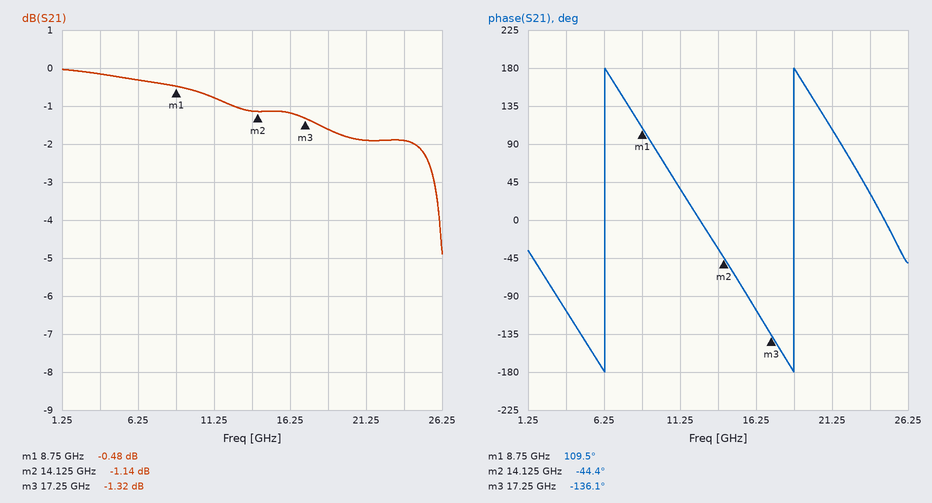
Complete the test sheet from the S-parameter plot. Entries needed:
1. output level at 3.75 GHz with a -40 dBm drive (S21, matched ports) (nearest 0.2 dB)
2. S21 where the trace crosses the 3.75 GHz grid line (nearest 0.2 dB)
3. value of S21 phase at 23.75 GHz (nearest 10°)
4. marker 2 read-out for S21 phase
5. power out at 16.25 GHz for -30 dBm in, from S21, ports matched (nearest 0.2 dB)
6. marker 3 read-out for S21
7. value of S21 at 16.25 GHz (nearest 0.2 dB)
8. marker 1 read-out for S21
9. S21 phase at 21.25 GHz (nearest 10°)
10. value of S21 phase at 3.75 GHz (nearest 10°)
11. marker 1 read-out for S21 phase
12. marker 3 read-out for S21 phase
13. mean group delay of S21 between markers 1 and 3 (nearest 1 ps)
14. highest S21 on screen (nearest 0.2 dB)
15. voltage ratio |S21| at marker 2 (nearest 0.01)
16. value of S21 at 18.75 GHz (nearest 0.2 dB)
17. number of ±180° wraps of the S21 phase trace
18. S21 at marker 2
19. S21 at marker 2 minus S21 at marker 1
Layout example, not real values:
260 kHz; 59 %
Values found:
-40.2 dBm; -0.2 dB; 30°; -44.4°; -31.2 dBm; -1.32 dB; -1.2 dB; -0.48 dB; 110°; -110°; 109.5°; -136.1°; 80 ps; 0.0 dB; 0.88; -1.6 dB; 2; -1.14 dB; -0.66 dB
